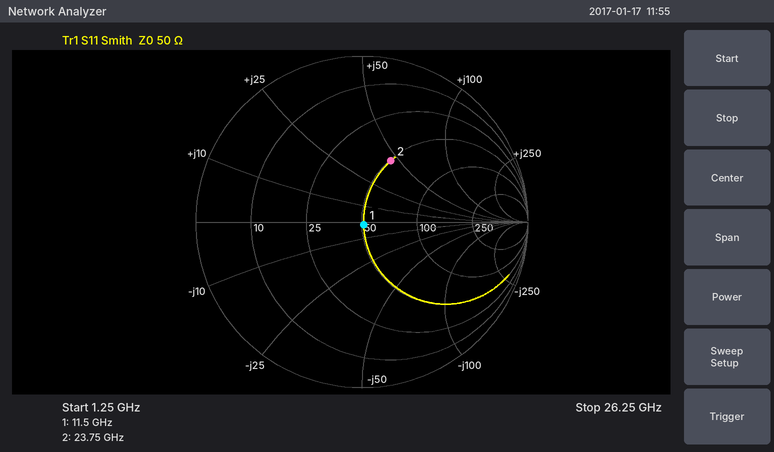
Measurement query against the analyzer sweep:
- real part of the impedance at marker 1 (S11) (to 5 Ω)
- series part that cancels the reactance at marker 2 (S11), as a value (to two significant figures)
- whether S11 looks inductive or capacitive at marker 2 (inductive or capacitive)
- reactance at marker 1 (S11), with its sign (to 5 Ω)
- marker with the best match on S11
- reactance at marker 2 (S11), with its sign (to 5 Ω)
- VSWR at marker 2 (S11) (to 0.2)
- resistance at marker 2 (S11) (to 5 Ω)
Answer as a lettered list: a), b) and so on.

a) 50 Ω
b) 150 fF
c) inductive
d) 0 Ω
e) marker 1
f) +45 Ω
g) 2.4
h) 50 Ω
